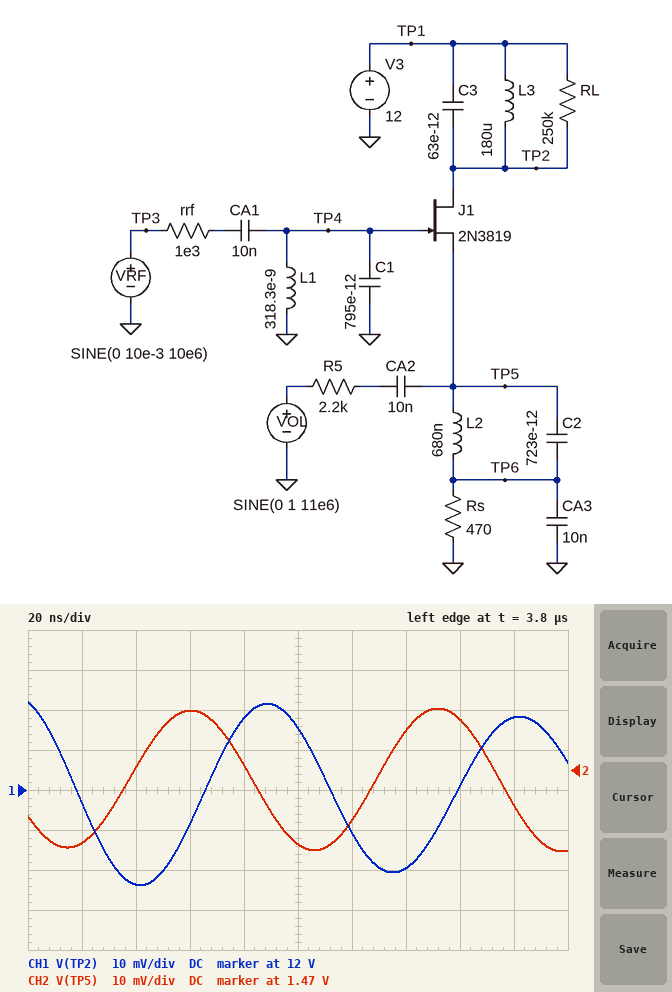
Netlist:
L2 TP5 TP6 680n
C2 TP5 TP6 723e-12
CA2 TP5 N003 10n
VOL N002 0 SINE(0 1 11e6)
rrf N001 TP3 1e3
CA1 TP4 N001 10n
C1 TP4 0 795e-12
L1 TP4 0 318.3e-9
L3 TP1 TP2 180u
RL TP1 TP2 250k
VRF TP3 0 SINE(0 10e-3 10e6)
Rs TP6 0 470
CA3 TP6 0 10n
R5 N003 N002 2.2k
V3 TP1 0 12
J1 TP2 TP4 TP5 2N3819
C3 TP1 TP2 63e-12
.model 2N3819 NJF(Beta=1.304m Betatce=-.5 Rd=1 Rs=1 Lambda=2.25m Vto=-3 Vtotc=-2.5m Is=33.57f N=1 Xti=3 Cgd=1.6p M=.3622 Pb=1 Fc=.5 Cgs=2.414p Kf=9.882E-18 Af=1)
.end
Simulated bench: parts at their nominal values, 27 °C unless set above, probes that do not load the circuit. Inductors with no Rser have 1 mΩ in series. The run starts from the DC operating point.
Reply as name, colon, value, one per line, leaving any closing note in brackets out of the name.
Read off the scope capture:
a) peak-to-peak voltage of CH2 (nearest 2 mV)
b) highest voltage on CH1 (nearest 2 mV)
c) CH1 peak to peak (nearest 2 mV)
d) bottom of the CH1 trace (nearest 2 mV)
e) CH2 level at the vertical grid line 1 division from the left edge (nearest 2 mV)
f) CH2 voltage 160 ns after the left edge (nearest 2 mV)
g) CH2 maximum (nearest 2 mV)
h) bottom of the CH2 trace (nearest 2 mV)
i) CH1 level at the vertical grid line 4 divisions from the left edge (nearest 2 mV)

peak-to-peak voltage of CH2: 36 mV
highest voltage on CH1: 12.022 V
CH1 peak to peak: 46 mV
bottom of the CH1 trace: 11.976 V
CH2 level at the vertical grid line 1 division from the left edge: 1.452 V
CH2 voltage 160 ns after the left edge: 1.482 V
CH2 maximum: 1.486 V
bottom of the CH2 trace: 1.450 V
CH1 level at the vertical grid line 4 divisions from the left edge: 12.018 V
